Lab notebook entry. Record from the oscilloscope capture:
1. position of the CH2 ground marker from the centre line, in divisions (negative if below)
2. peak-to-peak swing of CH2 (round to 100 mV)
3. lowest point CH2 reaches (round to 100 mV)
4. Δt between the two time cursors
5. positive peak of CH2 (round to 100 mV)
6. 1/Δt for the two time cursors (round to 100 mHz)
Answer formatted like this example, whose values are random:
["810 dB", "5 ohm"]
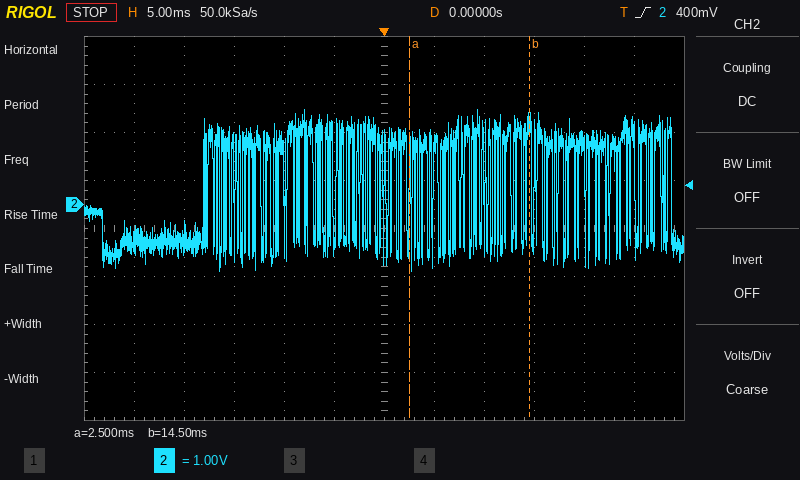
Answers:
["+0.5 div", "3.4 V", "-1.4 V", "12.0 ms", "2.0 V", "83.3 Hz"]
